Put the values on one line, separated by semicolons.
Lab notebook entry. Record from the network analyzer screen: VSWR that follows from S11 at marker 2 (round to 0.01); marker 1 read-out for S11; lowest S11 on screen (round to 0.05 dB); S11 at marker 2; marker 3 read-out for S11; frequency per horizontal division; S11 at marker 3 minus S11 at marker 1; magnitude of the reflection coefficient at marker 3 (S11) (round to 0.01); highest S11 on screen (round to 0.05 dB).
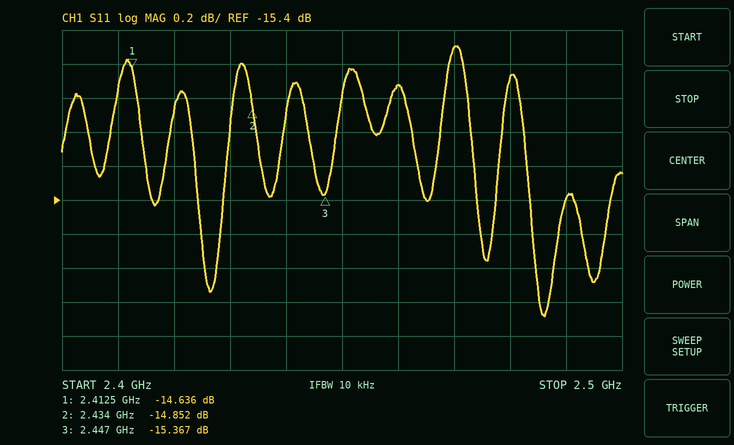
1.44; -14.636 dB; -16.10 dB; -14.852 dB; -15.367 dB; 10 MHz; -0.731 dB; 0.17; -14.50 dB
